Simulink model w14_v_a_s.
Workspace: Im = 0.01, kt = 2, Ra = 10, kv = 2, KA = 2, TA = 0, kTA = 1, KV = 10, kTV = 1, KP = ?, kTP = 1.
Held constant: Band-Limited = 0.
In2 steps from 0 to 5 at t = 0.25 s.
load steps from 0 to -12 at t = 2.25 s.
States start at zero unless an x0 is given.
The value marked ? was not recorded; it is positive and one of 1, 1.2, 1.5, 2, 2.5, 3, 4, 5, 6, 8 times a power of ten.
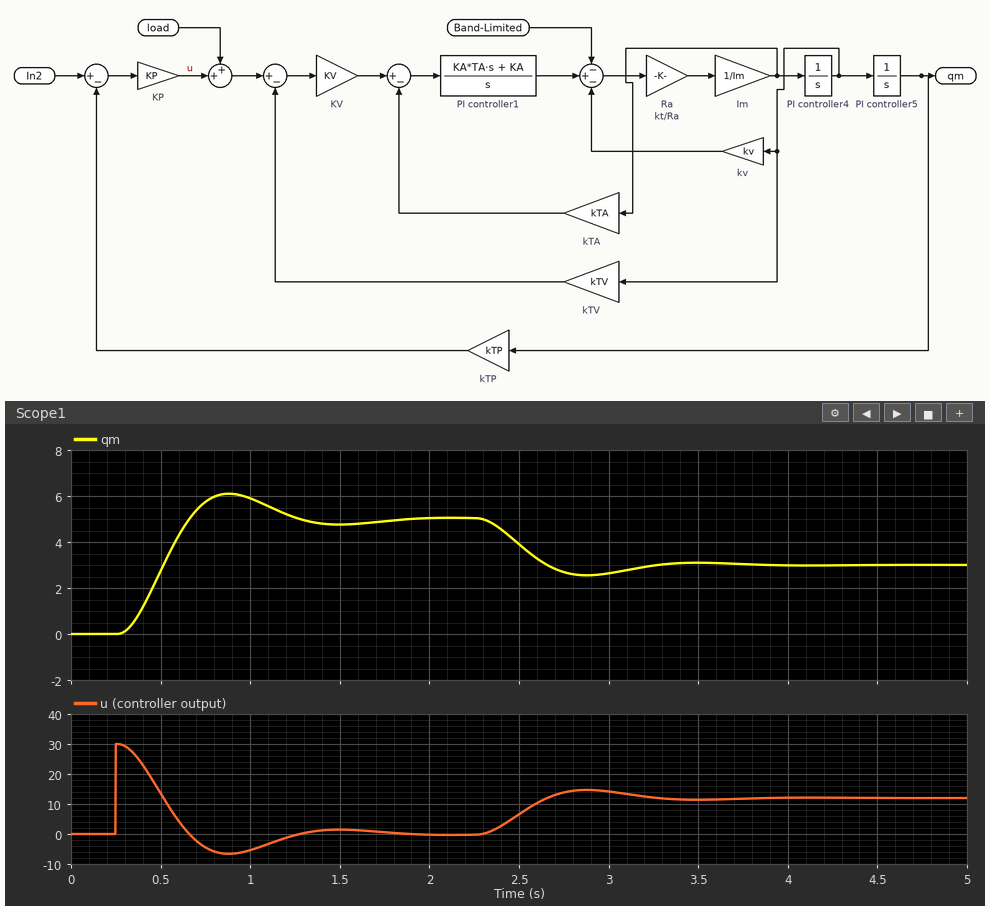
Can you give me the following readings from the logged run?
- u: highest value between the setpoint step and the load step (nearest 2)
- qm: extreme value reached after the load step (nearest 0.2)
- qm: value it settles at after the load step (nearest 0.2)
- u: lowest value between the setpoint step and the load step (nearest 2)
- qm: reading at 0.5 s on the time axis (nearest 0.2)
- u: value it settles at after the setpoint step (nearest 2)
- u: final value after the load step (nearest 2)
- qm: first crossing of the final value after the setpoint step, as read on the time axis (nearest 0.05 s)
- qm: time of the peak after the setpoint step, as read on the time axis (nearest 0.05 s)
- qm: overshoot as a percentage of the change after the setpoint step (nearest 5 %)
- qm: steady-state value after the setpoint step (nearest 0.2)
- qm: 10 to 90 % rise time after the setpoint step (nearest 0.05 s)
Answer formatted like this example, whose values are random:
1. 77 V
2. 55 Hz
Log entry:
1. 30
2. 2.6
3. 3.0
4. -6
5. 2.8
6. 0
7. 12
8. 0.65 s
9. 0.90 s
10. 20 %
11. 5.0
12. 0.25 s
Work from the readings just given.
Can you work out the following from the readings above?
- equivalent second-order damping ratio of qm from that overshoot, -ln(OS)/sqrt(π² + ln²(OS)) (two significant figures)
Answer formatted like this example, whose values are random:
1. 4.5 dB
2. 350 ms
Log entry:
1. 0.46
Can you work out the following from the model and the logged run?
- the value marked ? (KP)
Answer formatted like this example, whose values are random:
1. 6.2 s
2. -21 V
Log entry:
1. 6
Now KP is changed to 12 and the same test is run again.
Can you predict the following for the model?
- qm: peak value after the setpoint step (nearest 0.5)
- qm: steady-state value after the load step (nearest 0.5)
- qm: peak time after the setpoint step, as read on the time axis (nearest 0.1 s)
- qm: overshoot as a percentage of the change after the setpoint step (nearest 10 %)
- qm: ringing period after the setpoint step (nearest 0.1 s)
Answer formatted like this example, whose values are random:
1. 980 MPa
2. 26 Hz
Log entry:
1. 7.0
2. 4.0
3. 0.7 s
4. 40 %
5. 0.8 s
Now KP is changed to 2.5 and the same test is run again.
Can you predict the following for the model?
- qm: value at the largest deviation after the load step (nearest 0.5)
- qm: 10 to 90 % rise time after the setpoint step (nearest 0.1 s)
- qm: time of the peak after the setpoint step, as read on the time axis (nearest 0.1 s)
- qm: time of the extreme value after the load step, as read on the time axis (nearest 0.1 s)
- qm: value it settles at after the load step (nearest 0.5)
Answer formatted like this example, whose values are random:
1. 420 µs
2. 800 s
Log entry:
1. 0.0
2. 0.6 s
3. 1.5 s
4. 3.5 s
5. 0.0
